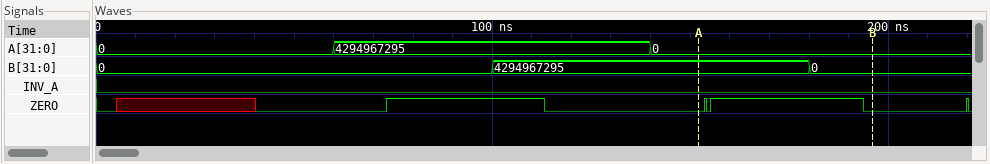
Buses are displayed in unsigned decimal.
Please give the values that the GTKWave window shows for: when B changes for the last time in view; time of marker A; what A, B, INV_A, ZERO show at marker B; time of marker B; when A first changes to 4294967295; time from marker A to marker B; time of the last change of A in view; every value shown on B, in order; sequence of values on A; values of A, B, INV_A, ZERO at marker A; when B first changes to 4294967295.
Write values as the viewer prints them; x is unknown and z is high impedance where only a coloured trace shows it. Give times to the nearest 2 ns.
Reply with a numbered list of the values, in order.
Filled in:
1. 180 ns
2. 152 ns
3. A=0, B=0, INV_A=0, ZERO=0
4. 196 ns
5. 60 ns
6. 44 ns
7. 140 ns
8. 0, 4294967295, 0
9. 0, 4294967295, 0
10. A=0, B=4294967295, INV_A=0, ZERO=0
11. 100 ns
